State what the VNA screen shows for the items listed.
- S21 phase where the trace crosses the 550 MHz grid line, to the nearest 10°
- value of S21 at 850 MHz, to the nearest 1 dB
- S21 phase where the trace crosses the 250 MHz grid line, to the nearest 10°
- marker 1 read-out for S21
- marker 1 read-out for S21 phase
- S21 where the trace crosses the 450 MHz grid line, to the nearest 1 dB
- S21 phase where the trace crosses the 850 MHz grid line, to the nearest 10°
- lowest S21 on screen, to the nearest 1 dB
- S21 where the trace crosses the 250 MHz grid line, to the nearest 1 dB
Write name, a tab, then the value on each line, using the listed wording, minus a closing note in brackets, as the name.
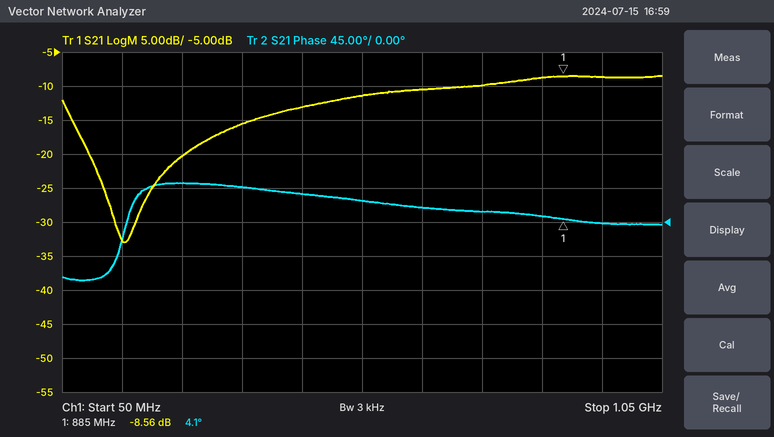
S21 phase where the trace crosses the 550 MHz grid line, to the nearest 10°	30°
value of S21 at 850 MHz, to the nearest 1 dB	-9 dB
S21 phase where the trace crosses the 250 MHz grid line, to the nearest 10°	50°
marker 1 read-out for S21	-8.56 dB
marker 1 read-out for S21 phase	4.1°
S21 where the trace crosses the 450 MHz grid line, to the nearest 1 dB	-13 dB
S21 phase where the trace crosses the 850 MHz grid line, to the nearest 10°	10°
lowest S21 on screen, to the nearest 1 dB	-33 dB
S21 where the trace crosses the 250 MHz grid line, to the nearest 1 dB	-20 dB
